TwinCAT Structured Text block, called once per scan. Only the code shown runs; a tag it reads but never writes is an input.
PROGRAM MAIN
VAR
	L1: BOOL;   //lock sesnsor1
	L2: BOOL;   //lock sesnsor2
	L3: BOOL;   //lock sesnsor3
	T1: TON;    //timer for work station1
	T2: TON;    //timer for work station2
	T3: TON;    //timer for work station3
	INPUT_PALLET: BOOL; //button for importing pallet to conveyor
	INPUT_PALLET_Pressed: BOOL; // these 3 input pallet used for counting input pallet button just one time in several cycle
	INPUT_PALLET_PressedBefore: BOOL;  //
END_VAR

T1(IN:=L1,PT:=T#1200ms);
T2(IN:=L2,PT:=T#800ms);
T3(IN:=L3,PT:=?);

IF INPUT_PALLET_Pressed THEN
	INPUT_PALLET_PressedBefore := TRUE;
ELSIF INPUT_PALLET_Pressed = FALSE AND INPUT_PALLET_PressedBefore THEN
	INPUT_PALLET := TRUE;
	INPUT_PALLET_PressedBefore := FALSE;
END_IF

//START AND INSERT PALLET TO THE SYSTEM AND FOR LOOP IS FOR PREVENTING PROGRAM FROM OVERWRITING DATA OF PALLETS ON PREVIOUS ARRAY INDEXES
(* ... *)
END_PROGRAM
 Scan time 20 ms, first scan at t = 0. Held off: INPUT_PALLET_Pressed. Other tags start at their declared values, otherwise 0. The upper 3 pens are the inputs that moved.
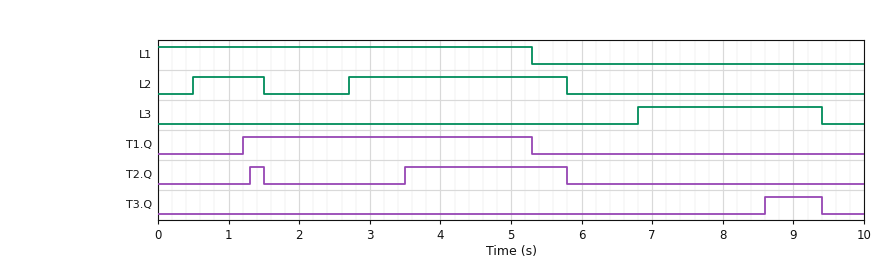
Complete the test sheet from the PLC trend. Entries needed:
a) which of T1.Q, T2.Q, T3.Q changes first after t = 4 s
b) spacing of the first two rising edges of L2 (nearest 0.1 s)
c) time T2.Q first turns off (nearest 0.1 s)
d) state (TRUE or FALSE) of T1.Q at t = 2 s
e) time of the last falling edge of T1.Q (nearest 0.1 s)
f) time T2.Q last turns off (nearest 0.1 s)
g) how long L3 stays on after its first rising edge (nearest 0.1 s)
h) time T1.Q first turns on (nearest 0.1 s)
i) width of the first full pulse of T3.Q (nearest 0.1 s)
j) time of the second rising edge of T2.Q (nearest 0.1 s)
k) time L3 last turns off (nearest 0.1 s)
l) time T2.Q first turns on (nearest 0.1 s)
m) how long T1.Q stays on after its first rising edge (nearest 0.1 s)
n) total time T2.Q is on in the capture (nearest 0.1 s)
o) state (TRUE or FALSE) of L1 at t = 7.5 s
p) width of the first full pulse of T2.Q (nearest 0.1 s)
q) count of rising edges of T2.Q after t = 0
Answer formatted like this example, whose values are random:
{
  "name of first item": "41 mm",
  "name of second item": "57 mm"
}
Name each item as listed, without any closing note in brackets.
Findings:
{
  "which of T1.Q, T2.Q, T3.Q changes first after t = 4 s": "T1.Q",
  "spacing of the first two rising edges of L2": "2.2 s",
  "time T2.Q first turns off": "1.5 s",
  "state (TRUE or FALSE) of T1.Q at t = 2 s": "TRUE",
  "time of the last falling edge of T1.Q": "5.3 s",
  "time T2.Q last turns off": "5.8 s",
  "how long L3 stays on after its first rising edge": "2.6 s",
  "time T1.Q first turns on": "1.2 s",
  "width of the first full pulse of T3.Q": "0.8 s",
  "time of the second rising edge of T2.Q": "3.5 s",
  "time L3 last turns off": "9.4 s",
  "time T2.Q first turns on": "1.3 s",
  "how long T1.Q stays on after its first rising edge": "4.1 s",
  "total time T2.Q is on in the capture": "2.5 s",
  "state (TRUE or FALSE) of L1 at t = 7.5 s": "FALSE",
  "width of the first full pulse of T2.Q": "0.2 s",
  "count of rising edges of T2.Q after t = 0": "2"
}
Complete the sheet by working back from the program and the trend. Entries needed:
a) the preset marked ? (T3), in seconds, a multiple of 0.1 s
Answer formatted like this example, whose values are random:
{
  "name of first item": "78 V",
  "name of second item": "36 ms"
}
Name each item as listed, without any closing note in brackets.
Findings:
{
  "the preset marked ? (T3), in seconds, a multiple of 0.1 s": "1.8 s"
}
